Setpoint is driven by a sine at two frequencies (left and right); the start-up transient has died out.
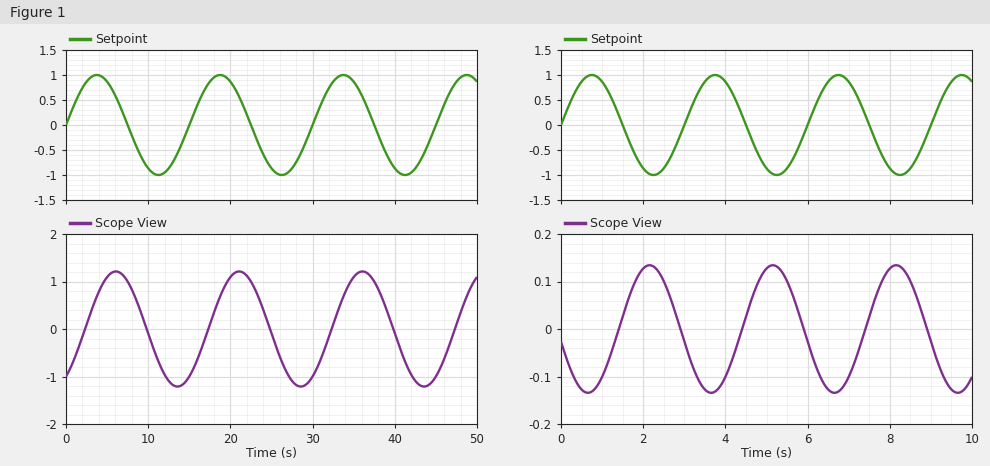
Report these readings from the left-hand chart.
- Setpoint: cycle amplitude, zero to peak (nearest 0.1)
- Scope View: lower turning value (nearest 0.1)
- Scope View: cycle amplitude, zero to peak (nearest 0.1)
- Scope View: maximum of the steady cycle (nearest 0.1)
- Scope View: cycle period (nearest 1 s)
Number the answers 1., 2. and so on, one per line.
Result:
1. 1.0
2. -1.2
3. 1.2
4. 1.2
5. 15 s
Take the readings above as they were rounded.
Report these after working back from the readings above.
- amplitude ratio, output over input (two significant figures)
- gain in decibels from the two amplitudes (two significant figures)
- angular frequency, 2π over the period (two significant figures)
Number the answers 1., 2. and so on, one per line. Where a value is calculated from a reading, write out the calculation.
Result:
1. 1.2 / 1 = 1.2
2. 20 log10(1.2 / 1) = 1.6 dB
3. 2π / 15 = 0.42 rad/s
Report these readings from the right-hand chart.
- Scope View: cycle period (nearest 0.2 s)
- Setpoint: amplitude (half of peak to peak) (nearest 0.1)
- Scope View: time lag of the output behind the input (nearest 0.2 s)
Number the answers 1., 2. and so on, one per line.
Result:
1. 3.0 s
2. 1.0
3. 1.4 s
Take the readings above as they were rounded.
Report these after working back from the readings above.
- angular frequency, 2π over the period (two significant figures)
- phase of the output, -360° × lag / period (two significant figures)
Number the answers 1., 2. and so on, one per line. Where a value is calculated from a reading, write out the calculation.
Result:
1. 2π / 3 = 2.1 rad/s
2. -360 × 1.4 / 3 = -170°
